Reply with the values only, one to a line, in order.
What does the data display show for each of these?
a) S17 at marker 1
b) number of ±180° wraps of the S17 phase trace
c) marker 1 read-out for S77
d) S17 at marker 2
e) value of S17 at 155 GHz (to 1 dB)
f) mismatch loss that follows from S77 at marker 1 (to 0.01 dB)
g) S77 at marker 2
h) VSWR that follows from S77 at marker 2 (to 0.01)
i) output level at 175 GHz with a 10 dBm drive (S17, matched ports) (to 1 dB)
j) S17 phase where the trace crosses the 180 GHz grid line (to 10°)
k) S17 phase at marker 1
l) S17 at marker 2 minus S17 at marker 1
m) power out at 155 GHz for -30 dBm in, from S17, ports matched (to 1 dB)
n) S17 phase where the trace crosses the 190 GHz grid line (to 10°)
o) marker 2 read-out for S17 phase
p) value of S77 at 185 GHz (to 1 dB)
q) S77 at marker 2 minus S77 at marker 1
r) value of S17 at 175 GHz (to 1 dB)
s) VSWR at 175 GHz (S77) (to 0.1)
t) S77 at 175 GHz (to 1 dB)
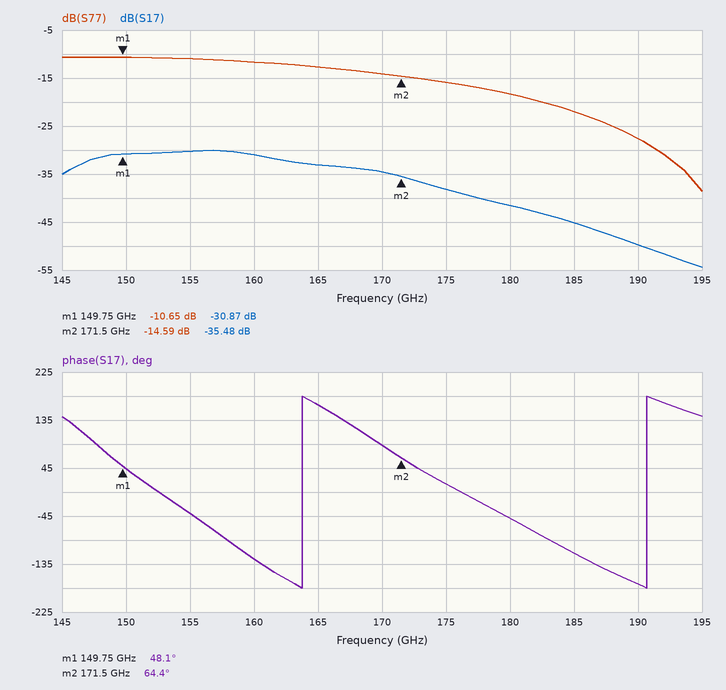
-30.87 dB
2
-10.65 dB
-35.48 dB
-30 dB
0.39 dB
-14.59 dB
1.46
-28 dBm
-50°
48.1°
-4.61 dB
-60 dBm
-170°
64.4°
-22 dB
-3.94 dB
-38 dB
1.4
-16 dB
